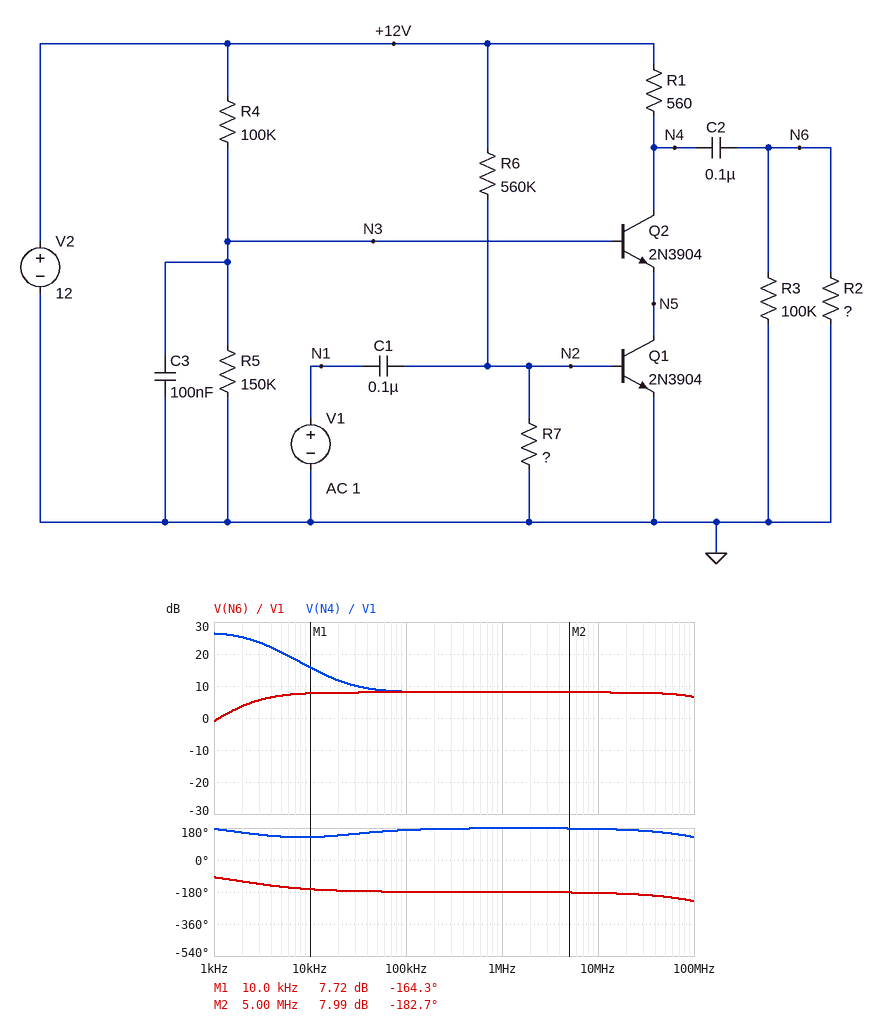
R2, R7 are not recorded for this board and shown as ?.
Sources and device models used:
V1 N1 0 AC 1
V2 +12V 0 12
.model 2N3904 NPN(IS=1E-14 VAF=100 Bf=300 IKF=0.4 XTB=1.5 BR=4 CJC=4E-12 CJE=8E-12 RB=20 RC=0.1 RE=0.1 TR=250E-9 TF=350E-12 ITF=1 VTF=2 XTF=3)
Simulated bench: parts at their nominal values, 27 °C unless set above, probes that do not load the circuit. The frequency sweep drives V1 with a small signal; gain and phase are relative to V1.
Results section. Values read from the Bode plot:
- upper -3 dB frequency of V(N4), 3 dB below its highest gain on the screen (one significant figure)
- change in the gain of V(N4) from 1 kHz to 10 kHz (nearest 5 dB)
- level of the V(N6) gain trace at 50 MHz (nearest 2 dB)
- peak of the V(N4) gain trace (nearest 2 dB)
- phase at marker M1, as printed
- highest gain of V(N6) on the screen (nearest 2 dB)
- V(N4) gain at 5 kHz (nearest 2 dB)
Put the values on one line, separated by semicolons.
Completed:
3 kHz; -10 dB; 8 dB; 26 dB; -164.3 deg; 8 dB; 20 dB
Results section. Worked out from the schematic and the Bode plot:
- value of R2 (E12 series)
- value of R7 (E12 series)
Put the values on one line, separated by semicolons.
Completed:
68 Ω; 39 kΩ
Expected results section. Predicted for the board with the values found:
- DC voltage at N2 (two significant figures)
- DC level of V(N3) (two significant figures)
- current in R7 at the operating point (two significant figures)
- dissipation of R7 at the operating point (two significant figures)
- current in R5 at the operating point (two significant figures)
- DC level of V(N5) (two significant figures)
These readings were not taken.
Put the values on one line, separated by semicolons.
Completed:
660 mV; 7.0 V; 17 µA; 11 µW; 47 µA; 6.3 V
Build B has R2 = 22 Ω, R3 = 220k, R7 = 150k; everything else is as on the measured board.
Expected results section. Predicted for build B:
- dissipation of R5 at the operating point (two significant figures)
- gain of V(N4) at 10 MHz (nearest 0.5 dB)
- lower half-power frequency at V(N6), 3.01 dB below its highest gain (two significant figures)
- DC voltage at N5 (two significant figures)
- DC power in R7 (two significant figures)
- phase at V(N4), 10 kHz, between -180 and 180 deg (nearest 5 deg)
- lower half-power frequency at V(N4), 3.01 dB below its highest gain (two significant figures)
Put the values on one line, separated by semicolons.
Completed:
260 µW; 11.5 dB; 3.0 kHz; 5.6 V; 3.2 µW; 120 deg; 600 Hz
